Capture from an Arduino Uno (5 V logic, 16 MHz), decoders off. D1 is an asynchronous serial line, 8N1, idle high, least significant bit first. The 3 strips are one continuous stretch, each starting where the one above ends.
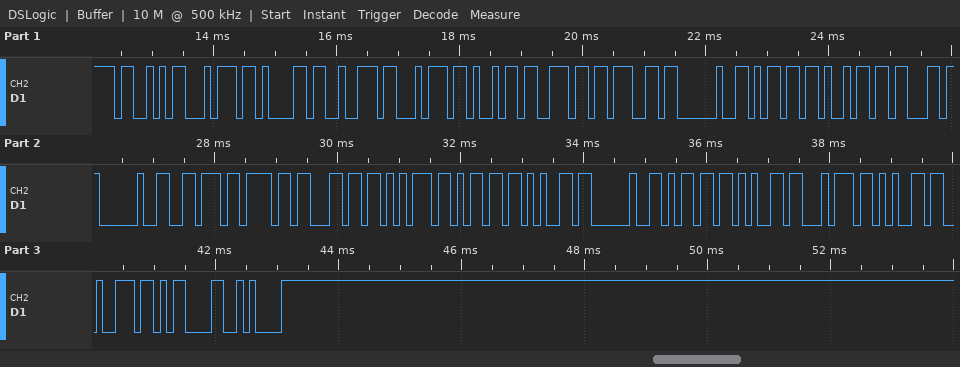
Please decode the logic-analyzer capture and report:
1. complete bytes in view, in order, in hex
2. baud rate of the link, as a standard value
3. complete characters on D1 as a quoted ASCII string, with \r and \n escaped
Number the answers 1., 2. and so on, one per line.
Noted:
1. 53 74 61 72 74 69 6E 67 20 6D 69 63 20 76 6F 6C 75 6D 65 20 6D 65 74 65 72 0D 0A
2. 9600 baud
3. "Starting mic volume meter\r\n"
